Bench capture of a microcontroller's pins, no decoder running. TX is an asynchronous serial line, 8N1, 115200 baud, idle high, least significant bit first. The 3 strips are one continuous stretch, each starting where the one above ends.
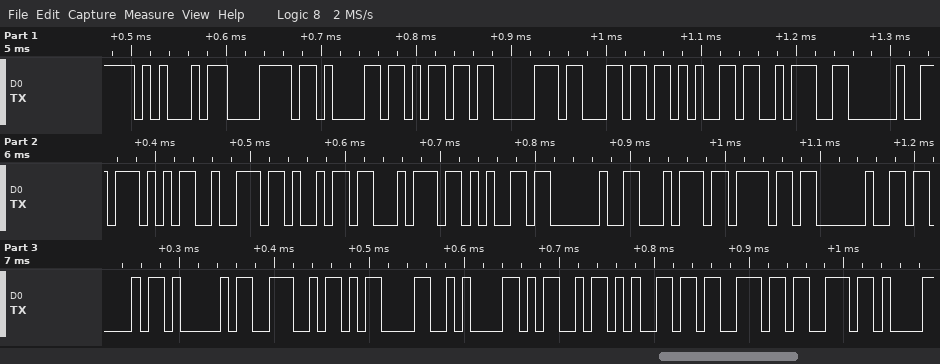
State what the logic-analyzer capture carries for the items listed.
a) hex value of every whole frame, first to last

45 78 61 6D 70 6C 65 3A 20 57 72 69 74 65 20 74 6F 20 43 41 4E 0D 0A 4D 65 73 73
